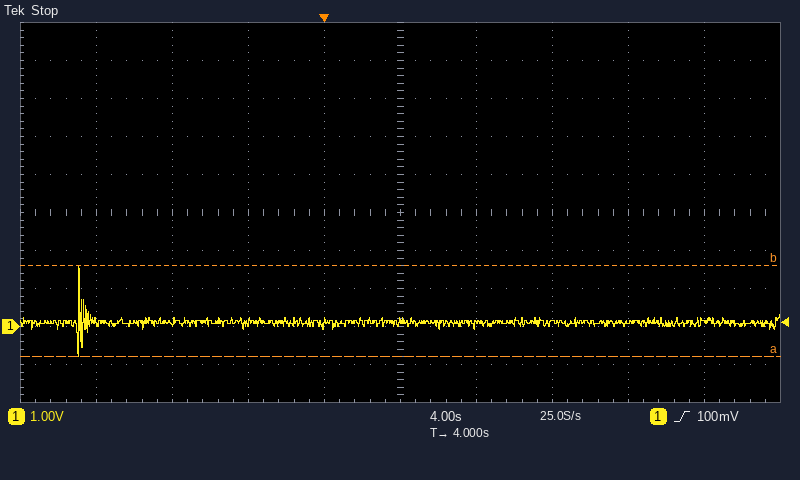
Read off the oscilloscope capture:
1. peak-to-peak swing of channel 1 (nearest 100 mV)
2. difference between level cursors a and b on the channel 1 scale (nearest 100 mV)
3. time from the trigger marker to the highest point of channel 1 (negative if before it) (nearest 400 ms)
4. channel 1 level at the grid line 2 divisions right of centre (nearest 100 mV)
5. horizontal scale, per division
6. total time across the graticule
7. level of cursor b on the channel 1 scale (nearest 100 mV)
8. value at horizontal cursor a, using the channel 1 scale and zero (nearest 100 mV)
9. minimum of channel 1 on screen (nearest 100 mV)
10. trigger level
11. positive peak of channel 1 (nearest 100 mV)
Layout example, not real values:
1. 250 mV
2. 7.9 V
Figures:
1. 2.4 V
2. 2.4 V
3. -12.8 s
4. 100 mV
5. 4 s
6. 40 s
7. 1.6 V
8. -800 mV
9. -800 mV
10. 100 mV
11. 1.6 V
